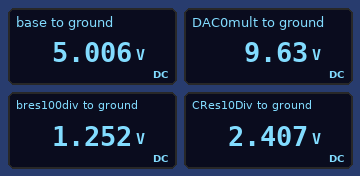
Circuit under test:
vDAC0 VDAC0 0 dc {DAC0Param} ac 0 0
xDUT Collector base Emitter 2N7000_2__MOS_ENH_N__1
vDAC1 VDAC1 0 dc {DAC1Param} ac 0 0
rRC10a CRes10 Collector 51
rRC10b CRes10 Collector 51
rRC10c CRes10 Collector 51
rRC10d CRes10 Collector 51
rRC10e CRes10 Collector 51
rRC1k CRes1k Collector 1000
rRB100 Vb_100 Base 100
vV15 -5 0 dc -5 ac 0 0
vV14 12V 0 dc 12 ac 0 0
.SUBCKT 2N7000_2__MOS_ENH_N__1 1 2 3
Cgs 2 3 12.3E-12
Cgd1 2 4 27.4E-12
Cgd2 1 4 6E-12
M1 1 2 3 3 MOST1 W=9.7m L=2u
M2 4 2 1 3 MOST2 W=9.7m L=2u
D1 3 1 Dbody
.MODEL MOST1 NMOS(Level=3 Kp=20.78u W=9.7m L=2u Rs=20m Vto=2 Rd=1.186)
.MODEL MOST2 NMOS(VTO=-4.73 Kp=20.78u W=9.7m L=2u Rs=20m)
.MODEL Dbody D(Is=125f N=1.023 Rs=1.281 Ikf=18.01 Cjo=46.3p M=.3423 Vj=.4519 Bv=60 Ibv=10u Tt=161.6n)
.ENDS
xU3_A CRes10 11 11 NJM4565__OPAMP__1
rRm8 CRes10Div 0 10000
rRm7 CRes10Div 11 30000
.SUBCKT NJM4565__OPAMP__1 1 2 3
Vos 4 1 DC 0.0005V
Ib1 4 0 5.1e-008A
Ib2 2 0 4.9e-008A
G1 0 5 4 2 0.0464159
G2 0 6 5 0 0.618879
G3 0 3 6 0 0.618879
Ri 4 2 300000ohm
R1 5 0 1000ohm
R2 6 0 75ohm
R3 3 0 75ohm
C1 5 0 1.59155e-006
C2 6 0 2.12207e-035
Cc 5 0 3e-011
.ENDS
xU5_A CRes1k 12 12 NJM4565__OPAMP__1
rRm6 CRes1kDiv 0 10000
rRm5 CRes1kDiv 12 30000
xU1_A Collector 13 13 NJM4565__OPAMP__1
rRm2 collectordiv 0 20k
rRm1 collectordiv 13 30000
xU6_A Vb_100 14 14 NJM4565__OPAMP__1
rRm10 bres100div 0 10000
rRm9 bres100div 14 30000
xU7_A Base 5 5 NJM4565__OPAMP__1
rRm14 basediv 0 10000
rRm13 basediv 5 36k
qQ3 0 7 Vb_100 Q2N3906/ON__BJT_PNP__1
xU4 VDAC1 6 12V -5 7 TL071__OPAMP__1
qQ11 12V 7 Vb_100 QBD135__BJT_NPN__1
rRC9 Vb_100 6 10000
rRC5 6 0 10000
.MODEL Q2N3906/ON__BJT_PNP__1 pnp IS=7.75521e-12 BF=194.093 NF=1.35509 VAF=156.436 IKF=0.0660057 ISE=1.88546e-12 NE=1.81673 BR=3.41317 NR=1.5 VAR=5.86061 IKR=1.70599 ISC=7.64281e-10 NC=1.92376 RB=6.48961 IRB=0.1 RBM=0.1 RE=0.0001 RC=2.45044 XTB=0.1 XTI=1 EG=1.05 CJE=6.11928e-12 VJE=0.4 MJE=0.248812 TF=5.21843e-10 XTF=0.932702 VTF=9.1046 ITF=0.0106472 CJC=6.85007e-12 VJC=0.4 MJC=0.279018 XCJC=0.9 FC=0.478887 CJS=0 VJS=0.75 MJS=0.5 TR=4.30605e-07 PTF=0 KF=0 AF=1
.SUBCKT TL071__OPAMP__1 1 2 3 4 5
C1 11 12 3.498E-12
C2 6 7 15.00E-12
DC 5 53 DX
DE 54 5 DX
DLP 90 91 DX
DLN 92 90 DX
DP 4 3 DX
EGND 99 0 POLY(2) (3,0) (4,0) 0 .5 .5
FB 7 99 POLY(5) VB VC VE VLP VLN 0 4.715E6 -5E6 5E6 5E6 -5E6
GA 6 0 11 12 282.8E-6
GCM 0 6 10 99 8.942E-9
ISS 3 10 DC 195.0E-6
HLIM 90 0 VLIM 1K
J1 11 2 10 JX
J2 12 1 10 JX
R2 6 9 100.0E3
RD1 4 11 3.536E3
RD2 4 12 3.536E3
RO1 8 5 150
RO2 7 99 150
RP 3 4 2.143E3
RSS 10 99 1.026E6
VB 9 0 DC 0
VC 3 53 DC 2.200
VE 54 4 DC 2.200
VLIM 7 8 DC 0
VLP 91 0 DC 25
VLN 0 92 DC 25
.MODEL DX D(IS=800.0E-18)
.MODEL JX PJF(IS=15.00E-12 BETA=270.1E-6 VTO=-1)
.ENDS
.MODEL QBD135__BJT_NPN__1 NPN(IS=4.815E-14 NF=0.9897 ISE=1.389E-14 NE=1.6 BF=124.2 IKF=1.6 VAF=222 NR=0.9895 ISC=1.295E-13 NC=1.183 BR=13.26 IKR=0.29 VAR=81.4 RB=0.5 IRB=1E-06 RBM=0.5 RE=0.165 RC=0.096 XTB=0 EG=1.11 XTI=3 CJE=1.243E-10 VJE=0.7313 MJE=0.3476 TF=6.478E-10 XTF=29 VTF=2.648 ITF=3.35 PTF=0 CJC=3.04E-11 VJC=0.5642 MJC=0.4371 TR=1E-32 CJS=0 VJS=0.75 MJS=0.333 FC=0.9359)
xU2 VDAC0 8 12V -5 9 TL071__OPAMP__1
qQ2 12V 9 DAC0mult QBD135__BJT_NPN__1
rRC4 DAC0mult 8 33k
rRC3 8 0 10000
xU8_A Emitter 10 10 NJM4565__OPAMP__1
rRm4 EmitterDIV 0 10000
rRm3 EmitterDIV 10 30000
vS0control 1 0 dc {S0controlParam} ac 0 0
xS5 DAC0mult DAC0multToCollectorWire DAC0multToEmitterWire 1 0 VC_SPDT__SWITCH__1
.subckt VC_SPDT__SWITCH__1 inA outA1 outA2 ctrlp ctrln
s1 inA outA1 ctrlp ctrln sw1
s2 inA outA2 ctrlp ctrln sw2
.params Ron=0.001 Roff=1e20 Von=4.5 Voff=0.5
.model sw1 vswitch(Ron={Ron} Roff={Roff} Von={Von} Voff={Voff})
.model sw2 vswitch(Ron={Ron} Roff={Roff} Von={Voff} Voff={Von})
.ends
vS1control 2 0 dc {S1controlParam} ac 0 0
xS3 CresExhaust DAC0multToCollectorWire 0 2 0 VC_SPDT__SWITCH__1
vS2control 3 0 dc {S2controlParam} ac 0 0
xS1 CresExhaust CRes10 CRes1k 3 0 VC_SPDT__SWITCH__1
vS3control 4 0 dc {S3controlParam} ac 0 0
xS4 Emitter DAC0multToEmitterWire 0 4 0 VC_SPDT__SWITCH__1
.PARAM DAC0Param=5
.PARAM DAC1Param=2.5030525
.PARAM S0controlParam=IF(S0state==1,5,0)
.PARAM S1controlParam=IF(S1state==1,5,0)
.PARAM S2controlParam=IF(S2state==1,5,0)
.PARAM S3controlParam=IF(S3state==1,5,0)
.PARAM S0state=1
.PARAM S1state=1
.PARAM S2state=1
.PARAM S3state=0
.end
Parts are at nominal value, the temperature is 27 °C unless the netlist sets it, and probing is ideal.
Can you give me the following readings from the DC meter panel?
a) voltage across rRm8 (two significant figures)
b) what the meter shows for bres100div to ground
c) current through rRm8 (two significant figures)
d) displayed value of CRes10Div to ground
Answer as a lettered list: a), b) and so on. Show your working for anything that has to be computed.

a) 2.407 V = 2.4 V
b) 1.252 V
c) (2.407 V) / 10 kΩ = 240 µA
d) 2.407 V
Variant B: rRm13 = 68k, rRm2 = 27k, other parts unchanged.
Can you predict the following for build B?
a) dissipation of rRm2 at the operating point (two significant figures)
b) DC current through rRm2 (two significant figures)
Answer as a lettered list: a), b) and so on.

a) 210 µW
b) 88 µA
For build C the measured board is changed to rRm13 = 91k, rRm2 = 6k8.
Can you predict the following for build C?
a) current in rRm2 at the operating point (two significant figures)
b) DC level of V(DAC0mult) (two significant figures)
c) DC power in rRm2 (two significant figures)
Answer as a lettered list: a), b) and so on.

a) 140 µA
b) 9.6 V
c) 130 µW
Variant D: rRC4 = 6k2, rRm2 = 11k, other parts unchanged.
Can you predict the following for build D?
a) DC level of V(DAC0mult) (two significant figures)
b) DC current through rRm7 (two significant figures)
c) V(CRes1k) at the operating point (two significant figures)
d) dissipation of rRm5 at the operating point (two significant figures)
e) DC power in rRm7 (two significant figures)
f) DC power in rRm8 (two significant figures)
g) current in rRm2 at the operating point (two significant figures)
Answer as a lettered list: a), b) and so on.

a) 8.1 V
b) 200 µA
c) 3.5 V
d) 230 µW
e) 1.2 mW
f) 410 µW
g) 85 µA
